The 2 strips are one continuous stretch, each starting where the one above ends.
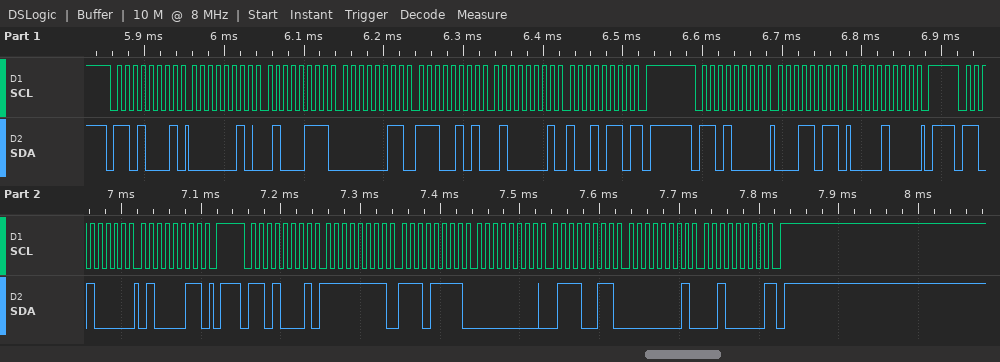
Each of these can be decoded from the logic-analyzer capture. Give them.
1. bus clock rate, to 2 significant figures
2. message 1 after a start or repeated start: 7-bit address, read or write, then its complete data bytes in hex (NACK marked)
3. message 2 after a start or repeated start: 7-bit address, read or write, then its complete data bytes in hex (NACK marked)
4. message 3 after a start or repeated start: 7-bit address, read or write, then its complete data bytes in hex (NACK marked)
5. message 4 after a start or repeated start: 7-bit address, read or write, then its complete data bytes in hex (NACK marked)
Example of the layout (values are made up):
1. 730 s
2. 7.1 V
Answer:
1. 100 kHz
2. 0x68 read: 02 47 03 E5 41 96 NACK
3. 0x68 write: 1B 08
4. 0x68 write: 43
5. 0x68 read: FF EF 00 73 01 20 NACK
